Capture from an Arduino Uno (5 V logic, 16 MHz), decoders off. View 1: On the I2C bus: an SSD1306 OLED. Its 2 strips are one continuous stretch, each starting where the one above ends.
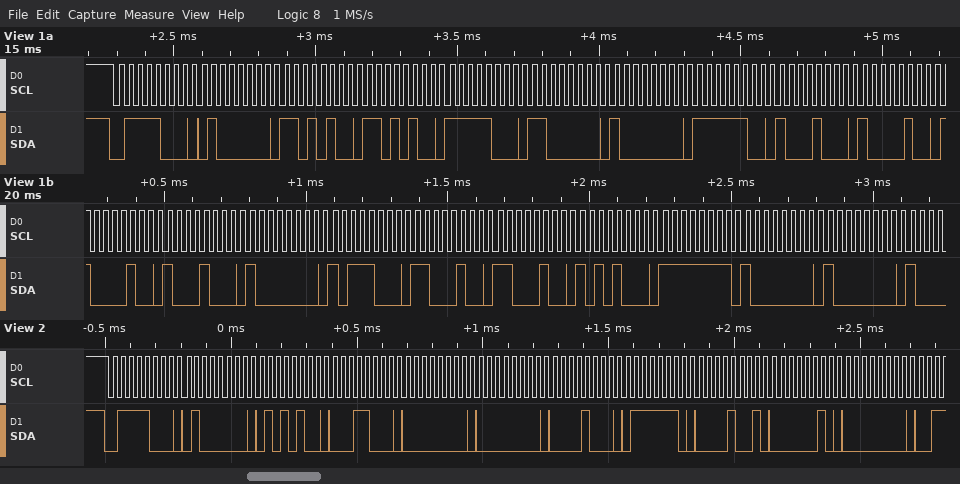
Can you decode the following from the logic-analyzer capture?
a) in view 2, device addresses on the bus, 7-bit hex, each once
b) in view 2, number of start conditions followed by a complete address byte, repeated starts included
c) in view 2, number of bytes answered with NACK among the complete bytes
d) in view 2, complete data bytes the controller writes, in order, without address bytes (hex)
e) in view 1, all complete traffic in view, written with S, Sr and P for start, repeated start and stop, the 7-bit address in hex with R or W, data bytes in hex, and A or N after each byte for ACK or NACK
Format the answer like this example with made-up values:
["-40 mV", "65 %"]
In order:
["0x3C", "1", "0", "40 54 18 00 00 08 7E 09 02 00", "S 3CW A 40 A D4 A D4 A F8 A C0 A 80 A FC A 88 A 84 A 84 A 88 A 80 A B8 A C4 A C4 A A8 A FF A 80 A 80 A"]
